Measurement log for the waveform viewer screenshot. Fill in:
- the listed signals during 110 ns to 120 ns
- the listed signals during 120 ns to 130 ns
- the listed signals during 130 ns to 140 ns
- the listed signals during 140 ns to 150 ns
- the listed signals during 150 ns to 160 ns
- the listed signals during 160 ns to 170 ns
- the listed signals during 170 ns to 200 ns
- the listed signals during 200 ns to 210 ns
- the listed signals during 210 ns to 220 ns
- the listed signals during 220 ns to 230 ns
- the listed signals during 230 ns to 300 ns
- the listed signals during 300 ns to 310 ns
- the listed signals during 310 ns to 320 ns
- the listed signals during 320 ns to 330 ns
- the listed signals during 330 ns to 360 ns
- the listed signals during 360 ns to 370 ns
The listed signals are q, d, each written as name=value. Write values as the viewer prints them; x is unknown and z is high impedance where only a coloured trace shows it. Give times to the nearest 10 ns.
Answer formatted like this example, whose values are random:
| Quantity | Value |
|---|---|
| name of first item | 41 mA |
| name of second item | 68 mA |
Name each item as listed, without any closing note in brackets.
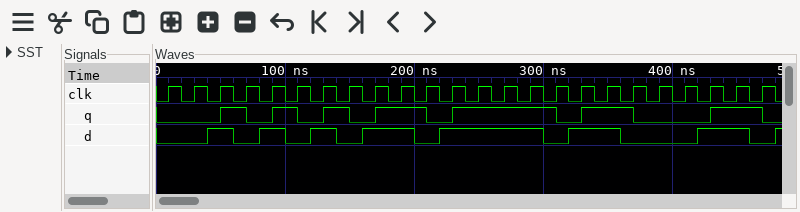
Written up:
| Quantity | Value |
|---|---|
| the listed signals during 110 ns to 120 ns | q=0, d=0 |
| the listed signals during 120 ns to 130 ns | q=0, d=1 |
| the listed signals during 130 ns to 140 ns | q=1, d=1 |
| the listed signals during 140 ns to 150 ns | q=1, d=0 |
| the listed signals during 150 ns to 160 ns | q=0, d=0 |
| the listed signals during 160 ns to 170 ns | q=0, d=1 |
| the listed signals during 170 ns to 200 ns | q=1, d=1 |
| the listed signals during 200 ns to 210 ns | q=1, d=0 |
| the listed signals during 210 ns to 220 ns | q=0, d=0 |
| the listed signals during 220 ns to 230 ns | q=0, d=1 |
| the listed signals during 230 ns to 300 ns | q=1, d=1 |
| the listed signals during 300 ns to 310 ns | q=1, d=0 |
| the listed signals during 310 ns to 320 ns | q=0, d=0 |
| the listed signals during 320 ns to 330 ns | q=0, d=1 |
| the listed signals during 330 ns to 360 ns | q=1, d=1 |
| the listed signals during 360 ns to 370 ns | q=1, d=0 |
